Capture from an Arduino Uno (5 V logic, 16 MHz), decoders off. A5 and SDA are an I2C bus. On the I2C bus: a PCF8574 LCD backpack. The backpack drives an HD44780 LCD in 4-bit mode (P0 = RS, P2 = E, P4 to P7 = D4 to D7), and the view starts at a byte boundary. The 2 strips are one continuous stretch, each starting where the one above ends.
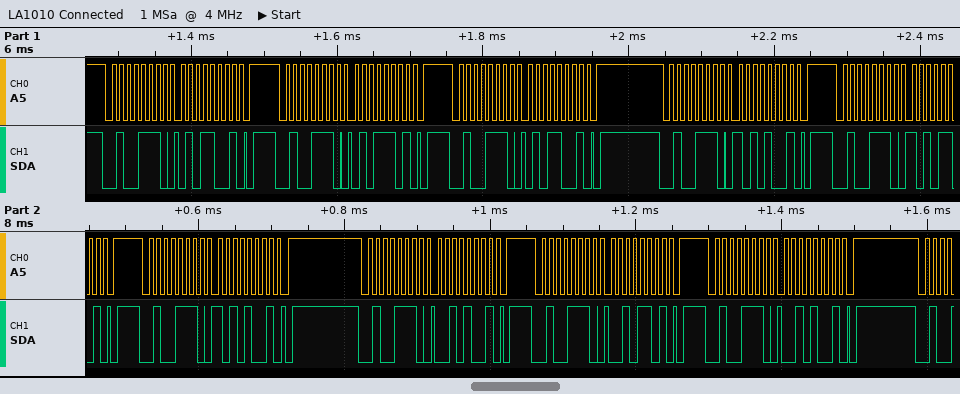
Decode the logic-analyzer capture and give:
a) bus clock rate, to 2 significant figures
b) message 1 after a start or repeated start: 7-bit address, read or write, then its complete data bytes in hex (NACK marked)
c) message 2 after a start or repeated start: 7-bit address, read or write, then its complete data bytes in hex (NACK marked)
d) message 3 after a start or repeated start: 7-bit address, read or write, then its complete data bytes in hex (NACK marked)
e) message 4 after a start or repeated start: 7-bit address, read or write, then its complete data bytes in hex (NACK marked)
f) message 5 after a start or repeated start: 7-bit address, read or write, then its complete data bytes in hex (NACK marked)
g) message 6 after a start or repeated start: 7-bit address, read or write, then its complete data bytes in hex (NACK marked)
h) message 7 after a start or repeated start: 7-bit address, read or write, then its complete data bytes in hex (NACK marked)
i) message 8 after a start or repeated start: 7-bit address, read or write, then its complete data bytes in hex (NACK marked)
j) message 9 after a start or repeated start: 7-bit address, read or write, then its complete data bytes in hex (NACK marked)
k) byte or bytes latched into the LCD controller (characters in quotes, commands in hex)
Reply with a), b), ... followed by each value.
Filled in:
a) 100 kHz
b) 0x27 write: 59
c) 0x27 write: 5D
d) 0x27 write: 59
e) 0x27 write: A9
f) 0x27 write: AD
g) 0x27 write: A9
h) 0x27 write: 29
i) 0x27 write: 2D
j) 0x27 write: 29
k) 'Z'
